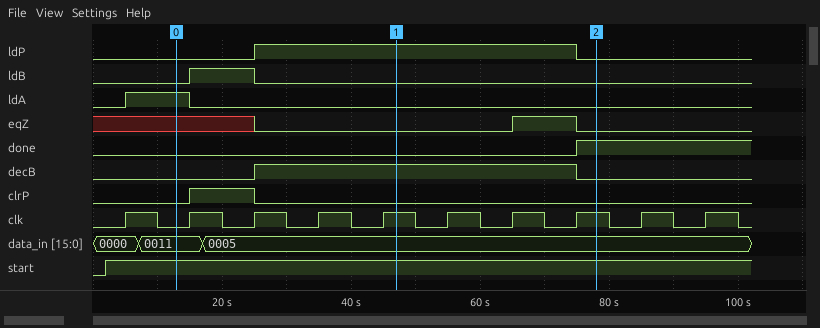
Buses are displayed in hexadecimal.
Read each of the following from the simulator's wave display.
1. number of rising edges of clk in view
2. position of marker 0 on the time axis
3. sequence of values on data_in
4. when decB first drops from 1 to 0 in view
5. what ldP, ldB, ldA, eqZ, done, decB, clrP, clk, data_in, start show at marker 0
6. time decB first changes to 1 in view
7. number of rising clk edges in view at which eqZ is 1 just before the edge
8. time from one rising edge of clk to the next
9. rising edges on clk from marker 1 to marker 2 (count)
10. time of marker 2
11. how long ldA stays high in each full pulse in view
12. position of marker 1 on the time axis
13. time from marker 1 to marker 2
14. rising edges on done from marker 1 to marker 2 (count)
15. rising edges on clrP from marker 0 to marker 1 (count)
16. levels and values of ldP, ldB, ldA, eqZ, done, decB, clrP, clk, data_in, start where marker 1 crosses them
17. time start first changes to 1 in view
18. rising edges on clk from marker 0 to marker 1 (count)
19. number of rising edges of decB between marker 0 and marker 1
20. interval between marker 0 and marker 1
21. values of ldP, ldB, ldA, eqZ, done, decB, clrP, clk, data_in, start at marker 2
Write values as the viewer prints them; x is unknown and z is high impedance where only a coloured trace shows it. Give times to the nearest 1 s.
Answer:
10
13 s
0000, 0011, 0005
75 s
ldP=0, ldB=0, ldA=1, eqZ=x, done=0, decB=0, clrP=0, clk=0, data_in=0011, start=1
25 s
1
10 s
3
78 s
10 s
47 s
31 s
1
1
ldP=1, ldB=0, ldA=0, eqZ=0, done=0, decB=1, clrP=0, clk=1, data_in=0005, start=1
2 s
4
1
34 s
ldP=0, ldB=0, ldA=0, eqZ=0, done=1, decB=0, clrP=0, clk=1, data_in=0005, start=1
